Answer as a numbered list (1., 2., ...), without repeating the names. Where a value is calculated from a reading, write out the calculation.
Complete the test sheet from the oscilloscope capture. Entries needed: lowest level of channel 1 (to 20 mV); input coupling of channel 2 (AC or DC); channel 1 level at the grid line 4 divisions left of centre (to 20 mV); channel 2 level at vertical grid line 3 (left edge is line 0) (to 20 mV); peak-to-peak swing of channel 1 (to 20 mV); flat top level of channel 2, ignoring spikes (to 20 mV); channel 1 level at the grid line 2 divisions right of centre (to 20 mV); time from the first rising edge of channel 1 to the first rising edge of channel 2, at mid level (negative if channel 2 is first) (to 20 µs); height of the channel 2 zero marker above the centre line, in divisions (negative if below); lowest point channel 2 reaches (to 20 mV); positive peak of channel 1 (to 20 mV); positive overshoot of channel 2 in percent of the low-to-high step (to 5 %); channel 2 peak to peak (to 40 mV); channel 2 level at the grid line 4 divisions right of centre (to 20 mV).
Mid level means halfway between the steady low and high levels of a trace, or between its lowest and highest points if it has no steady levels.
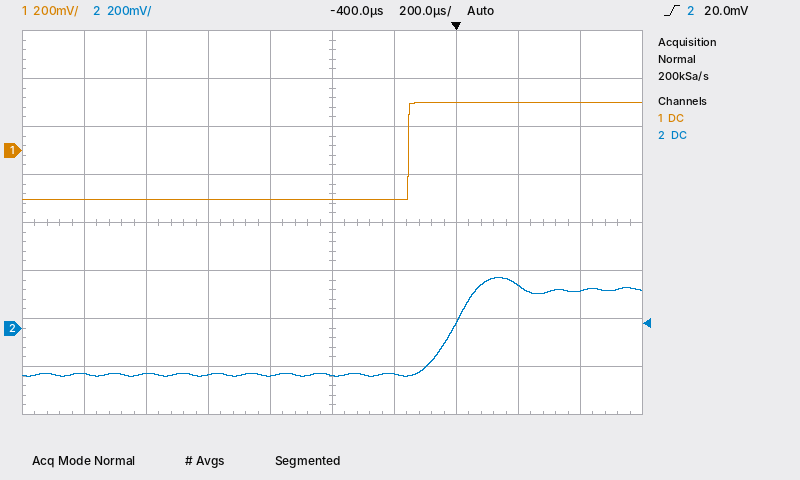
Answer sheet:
1. -200 mV
2. DC
3. -200 mV
4. -200 mV
5. 200 mV − (-200 mV) = 400 mV
6. 160 mV
7. 200 mV
8. +140 µs
9. -2.2 div
10. -200 mV
11. 200 mV
12. 15 %
13. 400 mV
14. 160 mV
